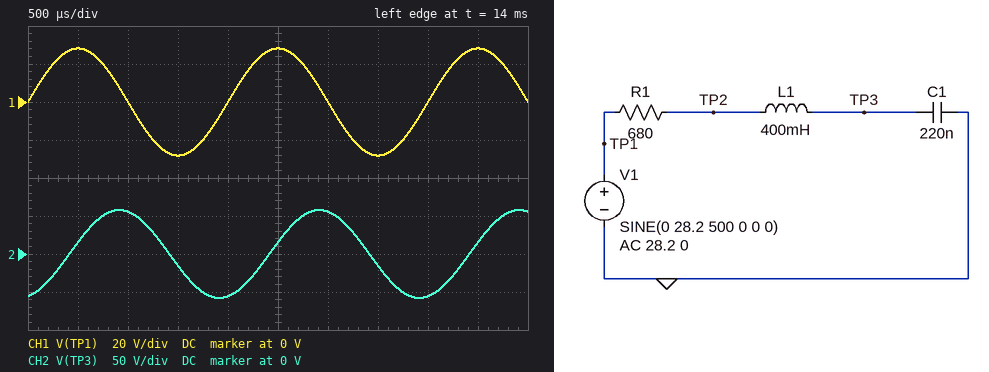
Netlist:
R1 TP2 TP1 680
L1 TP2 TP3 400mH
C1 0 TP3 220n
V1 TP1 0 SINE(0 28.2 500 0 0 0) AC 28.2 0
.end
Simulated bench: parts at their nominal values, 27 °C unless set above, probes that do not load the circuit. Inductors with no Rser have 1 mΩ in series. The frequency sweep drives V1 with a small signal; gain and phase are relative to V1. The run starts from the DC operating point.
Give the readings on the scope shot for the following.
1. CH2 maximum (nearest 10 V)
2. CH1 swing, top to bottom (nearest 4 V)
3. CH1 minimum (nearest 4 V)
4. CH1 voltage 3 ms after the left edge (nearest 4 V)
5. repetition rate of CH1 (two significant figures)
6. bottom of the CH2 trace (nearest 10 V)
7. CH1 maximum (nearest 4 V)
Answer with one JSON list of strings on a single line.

["60 V", "56 V", "-28 V", "0 V", "500 Hz", "-60 V", "28 V"]
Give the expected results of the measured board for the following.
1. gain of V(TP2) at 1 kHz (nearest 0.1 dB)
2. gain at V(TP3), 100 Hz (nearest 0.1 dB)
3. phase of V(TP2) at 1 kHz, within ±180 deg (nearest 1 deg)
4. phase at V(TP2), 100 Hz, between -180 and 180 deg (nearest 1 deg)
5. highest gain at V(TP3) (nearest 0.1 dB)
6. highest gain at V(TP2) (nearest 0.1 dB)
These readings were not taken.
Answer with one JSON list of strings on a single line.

["-0.6 dB", "0.3 dB", "21 deg", "-6 deg", "6.2 dB", "0 dB"]
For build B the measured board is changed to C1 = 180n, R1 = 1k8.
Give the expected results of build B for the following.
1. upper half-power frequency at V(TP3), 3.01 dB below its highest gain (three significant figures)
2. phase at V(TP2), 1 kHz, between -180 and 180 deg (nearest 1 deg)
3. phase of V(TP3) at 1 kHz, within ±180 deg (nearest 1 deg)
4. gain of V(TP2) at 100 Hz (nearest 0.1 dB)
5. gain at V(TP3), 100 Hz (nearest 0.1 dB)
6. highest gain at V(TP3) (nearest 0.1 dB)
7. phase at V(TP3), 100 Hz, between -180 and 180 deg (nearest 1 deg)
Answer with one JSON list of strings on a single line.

["659 Hz", "48 deg", "-132 deg", "-0.2 dB", "0.1 dB", "0.3 dB", "-12 deg"]
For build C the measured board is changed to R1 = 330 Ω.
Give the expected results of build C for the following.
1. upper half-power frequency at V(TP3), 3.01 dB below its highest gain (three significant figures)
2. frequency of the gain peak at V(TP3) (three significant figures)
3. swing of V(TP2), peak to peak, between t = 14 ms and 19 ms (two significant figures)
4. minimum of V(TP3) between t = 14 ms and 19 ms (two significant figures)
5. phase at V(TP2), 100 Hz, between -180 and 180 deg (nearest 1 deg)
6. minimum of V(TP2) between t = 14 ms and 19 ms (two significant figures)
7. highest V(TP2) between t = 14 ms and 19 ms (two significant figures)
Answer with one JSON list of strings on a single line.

["591 Hz", "528 Hz", "28 V", "-110 V", "-3 deg", "-14 V", "14 V"]
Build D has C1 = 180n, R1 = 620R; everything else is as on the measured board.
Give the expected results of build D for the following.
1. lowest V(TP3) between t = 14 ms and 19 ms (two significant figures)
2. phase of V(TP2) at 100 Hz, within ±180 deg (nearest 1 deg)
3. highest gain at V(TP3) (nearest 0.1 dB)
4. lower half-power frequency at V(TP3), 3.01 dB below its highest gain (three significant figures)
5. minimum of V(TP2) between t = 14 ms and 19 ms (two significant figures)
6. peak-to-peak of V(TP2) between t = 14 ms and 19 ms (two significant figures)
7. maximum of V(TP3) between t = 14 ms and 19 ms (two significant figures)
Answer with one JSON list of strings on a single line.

["-62 V", "-4 deg", "7.8 dB", "422 Hz", "-18 V", "36 V", "62 V"]
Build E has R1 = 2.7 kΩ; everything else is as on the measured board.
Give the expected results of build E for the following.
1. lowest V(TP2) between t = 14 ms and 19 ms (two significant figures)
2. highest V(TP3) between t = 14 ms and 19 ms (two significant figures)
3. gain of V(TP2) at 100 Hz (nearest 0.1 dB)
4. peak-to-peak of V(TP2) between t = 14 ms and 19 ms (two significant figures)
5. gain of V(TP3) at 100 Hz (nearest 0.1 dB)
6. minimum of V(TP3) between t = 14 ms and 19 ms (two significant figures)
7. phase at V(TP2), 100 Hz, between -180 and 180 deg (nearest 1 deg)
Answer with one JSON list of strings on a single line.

["-2.0 V", "15 V", "-0.6 dB", "4.0 V", "-0.3 dB", "-15 V", "-21 deg"]
